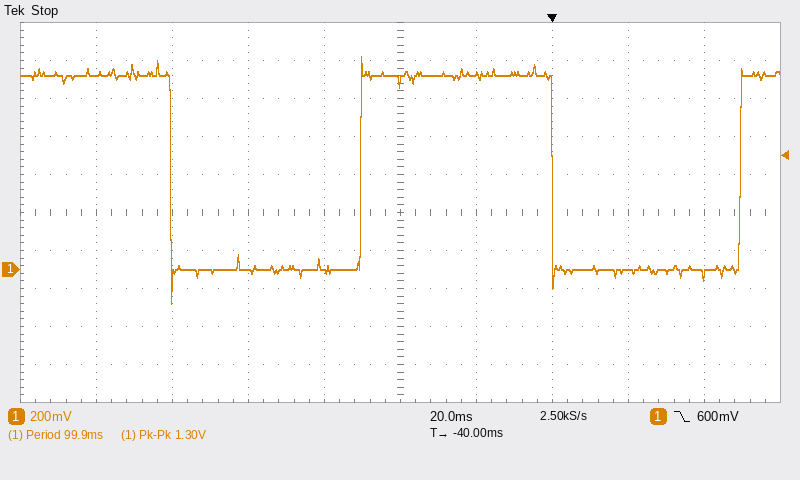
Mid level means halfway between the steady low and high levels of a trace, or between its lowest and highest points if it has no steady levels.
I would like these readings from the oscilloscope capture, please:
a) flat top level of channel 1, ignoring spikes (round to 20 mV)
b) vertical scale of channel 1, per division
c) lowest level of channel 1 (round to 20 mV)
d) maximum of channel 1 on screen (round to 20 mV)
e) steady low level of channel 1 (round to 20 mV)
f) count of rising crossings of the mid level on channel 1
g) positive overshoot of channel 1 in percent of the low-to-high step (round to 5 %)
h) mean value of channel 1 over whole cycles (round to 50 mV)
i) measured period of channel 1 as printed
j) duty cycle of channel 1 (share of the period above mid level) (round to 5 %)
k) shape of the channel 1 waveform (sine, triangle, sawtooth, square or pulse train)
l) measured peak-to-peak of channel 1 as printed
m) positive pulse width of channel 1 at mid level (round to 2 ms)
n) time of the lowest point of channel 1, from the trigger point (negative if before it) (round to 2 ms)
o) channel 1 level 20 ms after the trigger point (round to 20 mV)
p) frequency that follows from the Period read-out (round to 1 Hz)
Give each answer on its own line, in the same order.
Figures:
1.02 V
200 mV
-180 mV
1.12 V
0 mV
2
10 %
500 mV
99.9 ms
50 %
square
1.30 V
50 ms
-100 ms
0 mV
10 Hz
